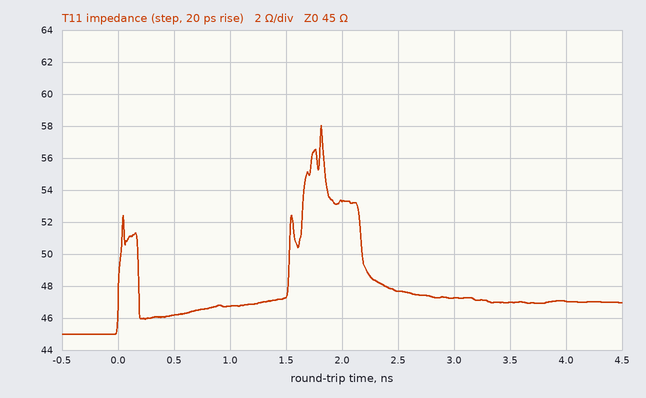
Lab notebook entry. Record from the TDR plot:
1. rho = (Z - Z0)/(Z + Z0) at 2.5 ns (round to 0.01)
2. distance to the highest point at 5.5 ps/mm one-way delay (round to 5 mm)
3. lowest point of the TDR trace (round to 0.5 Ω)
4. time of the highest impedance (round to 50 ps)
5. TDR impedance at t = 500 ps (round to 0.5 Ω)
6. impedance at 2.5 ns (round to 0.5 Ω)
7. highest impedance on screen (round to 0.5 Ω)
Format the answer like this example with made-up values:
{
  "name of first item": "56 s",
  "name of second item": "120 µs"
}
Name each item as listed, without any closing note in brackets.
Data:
{
  "rho = (Z - Z0)/(Z + Z0) at 2.5 ns": "+0.03",
  "distance to the highest point at 5.5 ps/mm one-way delay": "165 mm",
  "lowest point of the TDR trace": "45.0 Ω",
  "time of the highest impedance": "1.80 ns",
  "TDR impedance at t = 500 ps": "46.0 Ω",
  "impedance at 2.5 ns": "47.5 Ω",
  "highest impedance on screen": "58.0 Ω"
}
